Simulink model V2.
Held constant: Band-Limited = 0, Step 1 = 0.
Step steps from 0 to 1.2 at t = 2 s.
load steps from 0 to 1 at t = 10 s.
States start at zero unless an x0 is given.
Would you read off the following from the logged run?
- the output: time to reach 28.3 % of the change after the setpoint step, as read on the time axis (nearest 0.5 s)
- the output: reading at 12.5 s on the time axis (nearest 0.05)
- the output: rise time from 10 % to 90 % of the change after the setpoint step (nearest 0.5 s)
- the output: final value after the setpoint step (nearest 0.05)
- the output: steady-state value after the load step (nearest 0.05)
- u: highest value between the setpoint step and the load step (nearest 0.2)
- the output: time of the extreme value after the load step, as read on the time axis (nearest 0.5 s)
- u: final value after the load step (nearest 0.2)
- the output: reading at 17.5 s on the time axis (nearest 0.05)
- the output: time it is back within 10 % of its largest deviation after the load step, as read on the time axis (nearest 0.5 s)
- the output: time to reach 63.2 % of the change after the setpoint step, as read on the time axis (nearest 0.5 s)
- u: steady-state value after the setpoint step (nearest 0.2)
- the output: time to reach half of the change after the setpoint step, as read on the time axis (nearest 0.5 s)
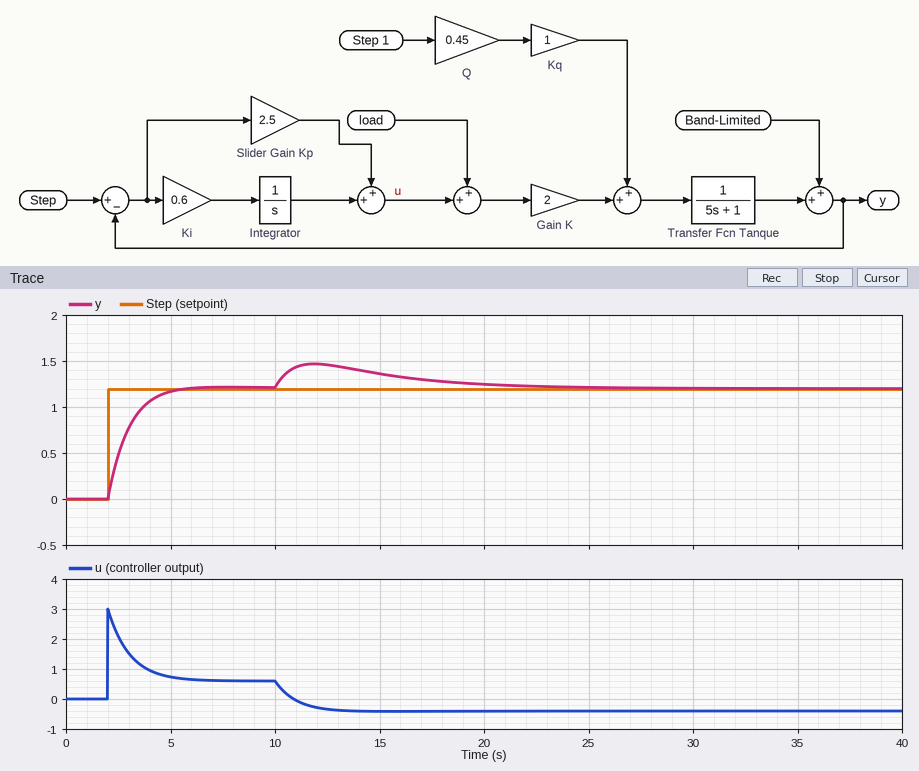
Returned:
2.5 s
1.45
2.0 s
1.20
1.20
3.0
12.0 s
-0.4
1.30
22.5 s
3.0 s
0.6
2.5 s
